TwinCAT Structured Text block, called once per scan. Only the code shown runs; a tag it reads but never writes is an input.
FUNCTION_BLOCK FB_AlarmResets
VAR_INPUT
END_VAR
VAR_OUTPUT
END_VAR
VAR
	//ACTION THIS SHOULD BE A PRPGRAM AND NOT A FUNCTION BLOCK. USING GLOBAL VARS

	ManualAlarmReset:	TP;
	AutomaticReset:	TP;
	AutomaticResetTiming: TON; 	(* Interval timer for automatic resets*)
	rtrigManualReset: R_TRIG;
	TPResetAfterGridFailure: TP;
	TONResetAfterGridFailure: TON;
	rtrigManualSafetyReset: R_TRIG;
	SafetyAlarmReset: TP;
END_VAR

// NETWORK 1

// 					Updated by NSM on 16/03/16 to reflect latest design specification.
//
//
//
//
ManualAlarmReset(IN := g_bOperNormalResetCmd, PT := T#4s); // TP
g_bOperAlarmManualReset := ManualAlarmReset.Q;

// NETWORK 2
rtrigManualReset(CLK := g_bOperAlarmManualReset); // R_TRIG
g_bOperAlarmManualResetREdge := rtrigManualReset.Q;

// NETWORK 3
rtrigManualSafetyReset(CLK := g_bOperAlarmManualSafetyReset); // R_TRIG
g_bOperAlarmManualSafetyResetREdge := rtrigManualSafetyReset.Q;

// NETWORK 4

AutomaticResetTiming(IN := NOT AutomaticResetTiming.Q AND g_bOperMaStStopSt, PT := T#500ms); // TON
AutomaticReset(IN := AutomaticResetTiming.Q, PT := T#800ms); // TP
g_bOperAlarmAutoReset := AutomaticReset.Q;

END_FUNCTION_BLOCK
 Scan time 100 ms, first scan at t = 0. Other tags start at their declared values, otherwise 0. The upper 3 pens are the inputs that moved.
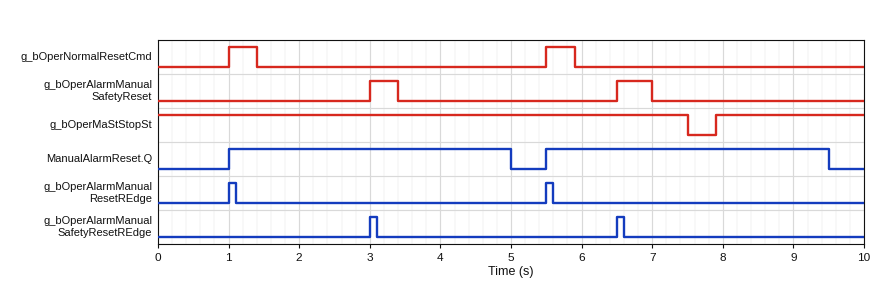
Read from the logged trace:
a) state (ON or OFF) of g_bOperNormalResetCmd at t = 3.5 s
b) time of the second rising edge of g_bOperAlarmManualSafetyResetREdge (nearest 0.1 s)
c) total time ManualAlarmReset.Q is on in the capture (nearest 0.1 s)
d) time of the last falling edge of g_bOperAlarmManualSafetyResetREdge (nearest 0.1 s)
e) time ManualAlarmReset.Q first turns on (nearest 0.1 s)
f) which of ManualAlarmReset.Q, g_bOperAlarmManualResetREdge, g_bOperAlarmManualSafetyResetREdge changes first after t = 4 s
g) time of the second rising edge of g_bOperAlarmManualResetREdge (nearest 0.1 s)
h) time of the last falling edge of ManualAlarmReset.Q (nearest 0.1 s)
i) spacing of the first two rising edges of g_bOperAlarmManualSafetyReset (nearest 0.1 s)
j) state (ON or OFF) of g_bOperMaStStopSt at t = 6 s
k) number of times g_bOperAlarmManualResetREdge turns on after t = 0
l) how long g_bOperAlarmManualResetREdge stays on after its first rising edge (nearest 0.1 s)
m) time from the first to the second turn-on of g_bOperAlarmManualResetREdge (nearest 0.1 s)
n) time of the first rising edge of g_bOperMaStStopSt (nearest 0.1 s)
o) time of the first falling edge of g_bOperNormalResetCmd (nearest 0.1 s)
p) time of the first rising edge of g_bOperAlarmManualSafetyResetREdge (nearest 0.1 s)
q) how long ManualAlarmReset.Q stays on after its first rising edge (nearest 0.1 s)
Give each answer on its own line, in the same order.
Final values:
OFF
6.5 s
8.0 s
6.6 s
1.0 s
ManualAlarmReset.Q
5.5 s
9.5 s
3.5 s
ON
2
0.1 s
4.5 s
7.9 s
1.4 s
3.0 s
4.0 s
